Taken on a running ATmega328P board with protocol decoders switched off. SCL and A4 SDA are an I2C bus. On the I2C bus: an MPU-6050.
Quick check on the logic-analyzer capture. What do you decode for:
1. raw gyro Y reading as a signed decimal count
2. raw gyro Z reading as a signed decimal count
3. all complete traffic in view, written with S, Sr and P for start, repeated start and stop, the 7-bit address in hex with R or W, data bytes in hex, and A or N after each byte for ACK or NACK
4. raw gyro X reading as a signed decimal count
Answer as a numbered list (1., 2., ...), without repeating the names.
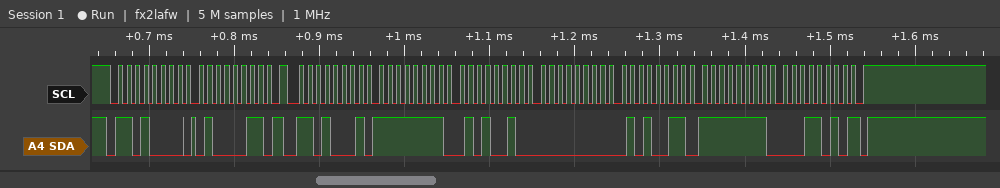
1. 83
2. -230
3. S 68W A 43 A Sr 68R A FF A 52 A 00 A 53 A FF A 1A N P
4. -174
